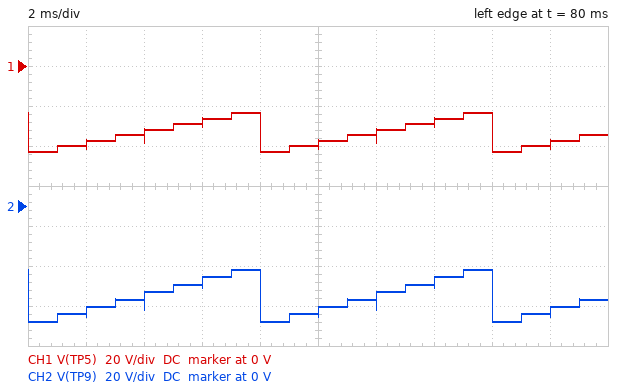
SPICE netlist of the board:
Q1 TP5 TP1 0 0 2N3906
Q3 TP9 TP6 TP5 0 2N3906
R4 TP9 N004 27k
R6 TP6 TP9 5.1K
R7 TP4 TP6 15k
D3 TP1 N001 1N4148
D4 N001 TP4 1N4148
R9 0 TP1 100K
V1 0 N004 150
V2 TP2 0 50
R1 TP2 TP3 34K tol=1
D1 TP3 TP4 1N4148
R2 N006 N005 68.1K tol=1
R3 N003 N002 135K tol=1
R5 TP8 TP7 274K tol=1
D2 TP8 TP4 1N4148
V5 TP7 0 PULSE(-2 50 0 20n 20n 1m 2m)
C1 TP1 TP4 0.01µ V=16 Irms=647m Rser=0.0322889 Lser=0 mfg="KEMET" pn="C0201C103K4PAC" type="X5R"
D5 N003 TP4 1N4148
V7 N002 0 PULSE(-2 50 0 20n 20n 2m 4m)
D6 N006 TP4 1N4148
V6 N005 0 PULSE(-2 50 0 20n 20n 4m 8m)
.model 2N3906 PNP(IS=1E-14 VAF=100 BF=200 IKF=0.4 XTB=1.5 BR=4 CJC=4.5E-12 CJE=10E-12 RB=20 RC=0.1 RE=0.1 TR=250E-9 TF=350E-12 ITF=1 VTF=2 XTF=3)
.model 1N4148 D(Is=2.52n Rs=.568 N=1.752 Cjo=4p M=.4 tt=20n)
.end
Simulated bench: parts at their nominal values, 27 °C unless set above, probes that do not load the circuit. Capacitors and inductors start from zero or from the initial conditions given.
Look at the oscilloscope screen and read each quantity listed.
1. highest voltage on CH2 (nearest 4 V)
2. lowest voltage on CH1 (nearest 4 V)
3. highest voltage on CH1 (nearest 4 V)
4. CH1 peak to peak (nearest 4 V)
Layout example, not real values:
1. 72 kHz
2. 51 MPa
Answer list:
1. -32 V
2. -44 V
3. -24 V
4. 20 V
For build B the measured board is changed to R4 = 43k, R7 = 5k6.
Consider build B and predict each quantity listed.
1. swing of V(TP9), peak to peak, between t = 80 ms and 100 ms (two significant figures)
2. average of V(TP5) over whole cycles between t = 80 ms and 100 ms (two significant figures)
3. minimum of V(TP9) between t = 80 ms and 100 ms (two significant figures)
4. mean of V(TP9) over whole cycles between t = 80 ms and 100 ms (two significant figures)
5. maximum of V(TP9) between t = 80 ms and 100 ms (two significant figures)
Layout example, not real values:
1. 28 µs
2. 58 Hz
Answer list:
1. 13 V
2. -13 V
3. -31 V
4. -24 V
5. -18 V
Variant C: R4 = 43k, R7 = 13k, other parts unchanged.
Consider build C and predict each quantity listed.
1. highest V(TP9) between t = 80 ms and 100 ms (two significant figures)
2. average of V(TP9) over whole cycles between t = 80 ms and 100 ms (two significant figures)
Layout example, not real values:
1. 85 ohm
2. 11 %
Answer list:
1. -29 V
2. -38 V
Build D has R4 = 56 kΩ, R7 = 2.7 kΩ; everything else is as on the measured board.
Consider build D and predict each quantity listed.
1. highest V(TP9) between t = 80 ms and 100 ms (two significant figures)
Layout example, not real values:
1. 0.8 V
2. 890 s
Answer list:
1. -13 V
